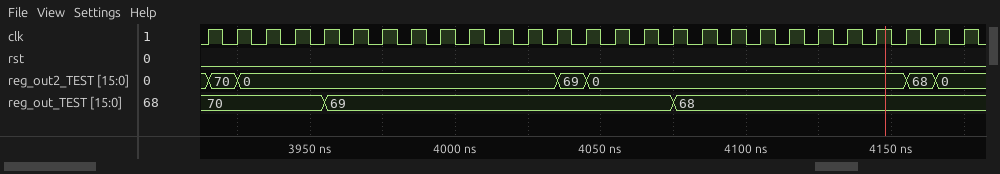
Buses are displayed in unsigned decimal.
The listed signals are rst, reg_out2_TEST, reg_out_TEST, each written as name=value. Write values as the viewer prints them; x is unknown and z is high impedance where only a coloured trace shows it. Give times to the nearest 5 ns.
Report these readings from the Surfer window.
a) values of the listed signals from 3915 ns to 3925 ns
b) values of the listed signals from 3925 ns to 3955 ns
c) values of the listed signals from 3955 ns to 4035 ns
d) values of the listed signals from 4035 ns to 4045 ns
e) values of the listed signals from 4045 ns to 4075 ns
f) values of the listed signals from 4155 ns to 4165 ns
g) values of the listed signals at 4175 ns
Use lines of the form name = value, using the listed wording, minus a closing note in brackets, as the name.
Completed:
values of the listed signals from 3915 ns to 3925 ns = rst=0, reg_out2_TEST=70, reg_out_TEST=70
values of the listed signals from 3925 ns to 3955 ns = rst=0, reg_out2_TEST=0, reg_out_TEST=70
values of the listed signals from 3955 ns to 4035 ns = rst=0, reg_out2_TEST=0, reg_out_TEST=69
values of the listed signals from 4035 ns to 4045 ns = rst=0, reg_out2_TEST=69, reg_out_TEST=69
values of the listed signals from 4045 ns to 4075 ns = rst=0, reg_out2_TEST=0, reg_out_TEST=69
values of the listed signals from 4155 ns to 4165 ns = rst=0, reg_out2_TEST=68, reg_out_TEST=68
values of the listed signals at 4175 ns = rst=0, reg_out2_TEST=0, reg_out_TEST=68
